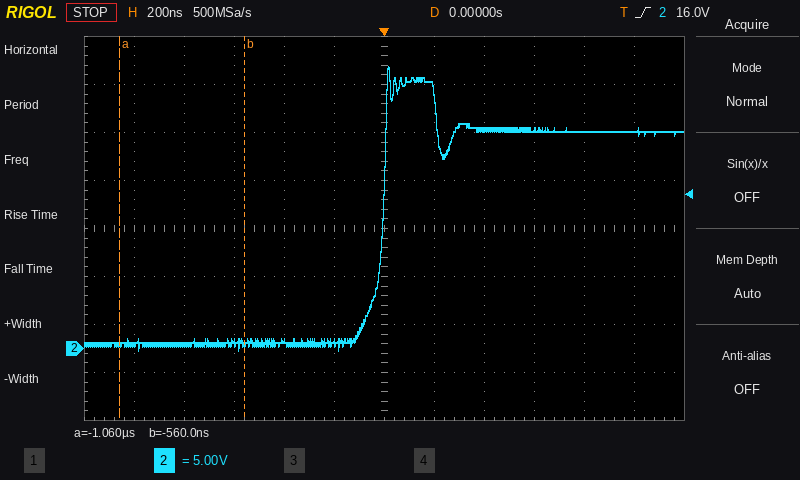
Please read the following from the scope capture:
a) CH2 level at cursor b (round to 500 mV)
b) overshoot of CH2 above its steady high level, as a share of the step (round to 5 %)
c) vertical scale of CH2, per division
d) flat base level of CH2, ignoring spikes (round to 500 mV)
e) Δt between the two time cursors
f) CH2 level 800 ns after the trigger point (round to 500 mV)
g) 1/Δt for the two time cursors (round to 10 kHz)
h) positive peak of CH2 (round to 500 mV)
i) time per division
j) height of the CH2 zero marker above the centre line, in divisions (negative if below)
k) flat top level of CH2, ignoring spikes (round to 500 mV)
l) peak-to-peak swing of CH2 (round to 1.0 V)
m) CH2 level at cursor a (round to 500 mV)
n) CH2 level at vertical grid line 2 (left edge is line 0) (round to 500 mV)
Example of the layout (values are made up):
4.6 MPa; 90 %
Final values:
500 mV; 30 %; 5 V; 500 mV; 500 ns; 22.5 V; 2.00 MHz; 29.5 V; 200 ns; -2.5 div; 22.5 V; 30.0 V; 500 mV; 500 mV
